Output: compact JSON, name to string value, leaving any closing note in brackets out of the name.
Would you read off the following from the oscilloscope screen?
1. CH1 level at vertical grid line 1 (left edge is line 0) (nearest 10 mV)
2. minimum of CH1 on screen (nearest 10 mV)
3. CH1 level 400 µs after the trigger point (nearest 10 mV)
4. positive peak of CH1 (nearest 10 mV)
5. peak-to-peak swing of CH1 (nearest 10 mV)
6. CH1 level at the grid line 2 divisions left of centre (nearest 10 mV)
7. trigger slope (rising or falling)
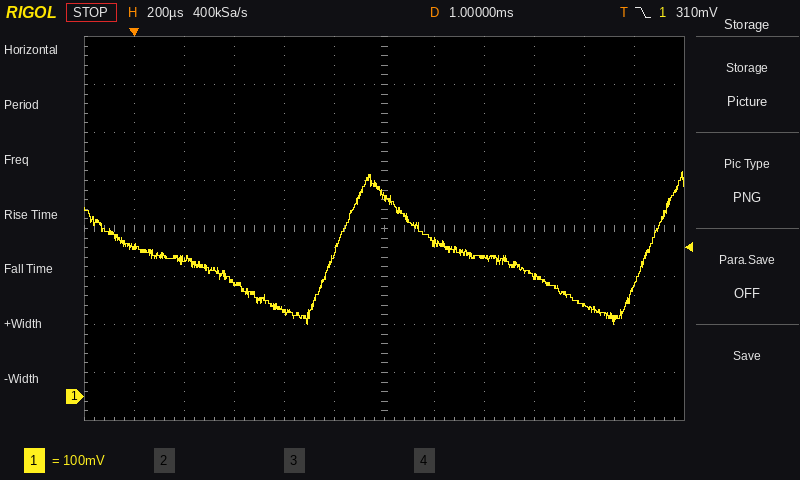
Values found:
{"CH1 level at vertical grid line 1 (left edge is line 0)": "310 mV", "minimum of CH1 on screen": "150 mV", "CH1 level 400 µs after the trigger point": "240 mV", "positive peak of CH1": "470 mV", "peak-to-peak swing of CH1": "320 mV", "CH1 level at the grid line 2 divisions left of centre": "180 mV", "trigger slope": "falling"}
